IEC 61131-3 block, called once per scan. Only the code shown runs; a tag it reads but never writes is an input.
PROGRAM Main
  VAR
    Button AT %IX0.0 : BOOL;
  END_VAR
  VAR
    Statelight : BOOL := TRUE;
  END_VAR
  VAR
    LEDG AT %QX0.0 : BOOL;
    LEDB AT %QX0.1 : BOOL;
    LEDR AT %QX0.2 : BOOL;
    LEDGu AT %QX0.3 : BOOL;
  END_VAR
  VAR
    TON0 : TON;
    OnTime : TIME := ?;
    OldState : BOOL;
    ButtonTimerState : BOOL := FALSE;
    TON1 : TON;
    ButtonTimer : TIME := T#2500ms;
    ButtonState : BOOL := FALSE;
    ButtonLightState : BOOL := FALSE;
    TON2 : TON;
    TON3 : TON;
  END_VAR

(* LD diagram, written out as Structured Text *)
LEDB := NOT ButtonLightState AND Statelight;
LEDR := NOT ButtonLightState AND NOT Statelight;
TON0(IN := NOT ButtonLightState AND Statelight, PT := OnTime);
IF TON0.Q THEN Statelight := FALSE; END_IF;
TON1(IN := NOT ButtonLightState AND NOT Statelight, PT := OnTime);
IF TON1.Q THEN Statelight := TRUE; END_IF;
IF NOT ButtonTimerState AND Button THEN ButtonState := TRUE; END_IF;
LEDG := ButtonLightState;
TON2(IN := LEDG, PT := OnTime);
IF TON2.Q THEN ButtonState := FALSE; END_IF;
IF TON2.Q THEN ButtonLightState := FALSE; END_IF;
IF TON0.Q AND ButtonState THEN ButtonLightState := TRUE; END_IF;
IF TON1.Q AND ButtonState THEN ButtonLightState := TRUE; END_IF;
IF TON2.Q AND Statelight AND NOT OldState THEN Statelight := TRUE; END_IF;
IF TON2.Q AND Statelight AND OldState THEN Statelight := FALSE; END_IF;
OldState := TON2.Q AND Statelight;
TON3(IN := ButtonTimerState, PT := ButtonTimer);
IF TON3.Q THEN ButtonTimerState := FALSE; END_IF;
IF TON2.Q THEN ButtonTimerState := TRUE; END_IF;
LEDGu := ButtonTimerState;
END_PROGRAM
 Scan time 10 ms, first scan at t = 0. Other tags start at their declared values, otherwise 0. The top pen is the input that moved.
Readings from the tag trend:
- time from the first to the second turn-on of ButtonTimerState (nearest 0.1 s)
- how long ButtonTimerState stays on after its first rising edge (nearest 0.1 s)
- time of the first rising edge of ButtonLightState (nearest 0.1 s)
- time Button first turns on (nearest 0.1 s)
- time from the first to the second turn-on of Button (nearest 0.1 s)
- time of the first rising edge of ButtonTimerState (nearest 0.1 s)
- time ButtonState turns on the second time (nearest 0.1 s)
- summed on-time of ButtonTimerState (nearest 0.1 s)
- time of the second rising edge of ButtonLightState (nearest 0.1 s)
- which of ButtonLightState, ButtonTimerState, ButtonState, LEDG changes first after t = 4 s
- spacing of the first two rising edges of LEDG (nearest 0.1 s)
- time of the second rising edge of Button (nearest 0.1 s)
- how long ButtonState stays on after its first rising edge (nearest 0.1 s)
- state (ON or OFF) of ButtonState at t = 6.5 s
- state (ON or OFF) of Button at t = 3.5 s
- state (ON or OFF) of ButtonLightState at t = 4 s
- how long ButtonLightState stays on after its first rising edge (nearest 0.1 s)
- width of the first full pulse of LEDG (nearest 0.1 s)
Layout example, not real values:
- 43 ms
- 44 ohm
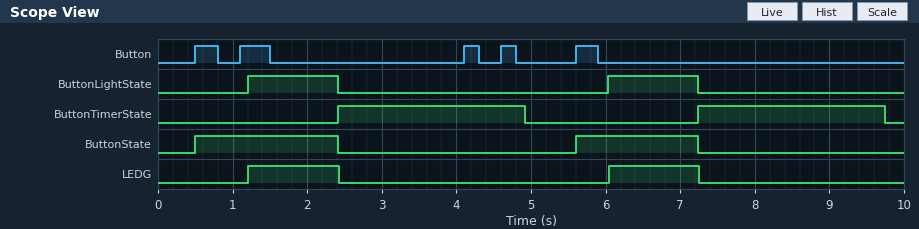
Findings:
- 4.8 s
- 2.5 s
- 1.2 s
- 0.5 s
- 0.6 s
- 2.4 s
- 5.6 s
- 5.0 s
- 6.0 s
- ButtonTimerState
- 4.8 s
- 1.1 s
- 1.9 s
- ON
- OFF
- OFF
- 1.2 s
- 1.2 s
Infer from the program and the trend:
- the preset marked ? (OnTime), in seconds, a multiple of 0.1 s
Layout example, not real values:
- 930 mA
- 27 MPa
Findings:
- 1.2 s
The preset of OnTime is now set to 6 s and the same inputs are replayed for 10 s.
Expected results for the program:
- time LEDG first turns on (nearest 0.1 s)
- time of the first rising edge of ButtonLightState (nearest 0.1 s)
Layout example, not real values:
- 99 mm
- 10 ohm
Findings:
- 6.0 s
- 6.0 s
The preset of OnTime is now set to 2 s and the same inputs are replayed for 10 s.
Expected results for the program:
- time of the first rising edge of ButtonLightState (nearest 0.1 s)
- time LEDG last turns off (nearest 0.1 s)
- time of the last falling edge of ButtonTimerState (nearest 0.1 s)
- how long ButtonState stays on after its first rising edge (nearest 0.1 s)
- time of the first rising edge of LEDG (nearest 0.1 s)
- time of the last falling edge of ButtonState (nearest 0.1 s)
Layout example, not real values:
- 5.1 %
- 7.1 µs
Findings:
- 2.0 s
- 4.0 s
- 6.5 s
- 3.5 s
- 2.0 s
- 4.0 s
